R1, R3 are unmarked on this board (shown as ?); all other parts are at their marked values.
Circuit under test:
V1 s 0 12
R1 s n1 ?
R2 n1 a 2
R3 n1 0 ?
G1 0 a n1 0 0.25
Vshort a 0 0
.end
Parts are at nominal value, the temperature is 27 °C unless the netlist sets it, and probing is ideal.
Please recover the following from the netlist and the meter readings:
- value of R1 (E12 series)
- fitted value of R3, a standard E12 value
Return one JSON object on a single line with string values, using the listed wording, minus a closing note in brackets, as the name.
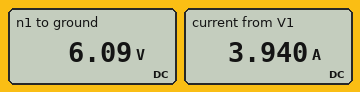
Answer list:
{"value of R1": "1.5 Ω", "fitted value of R3, a standard E12 value": "6.8 Ω"}
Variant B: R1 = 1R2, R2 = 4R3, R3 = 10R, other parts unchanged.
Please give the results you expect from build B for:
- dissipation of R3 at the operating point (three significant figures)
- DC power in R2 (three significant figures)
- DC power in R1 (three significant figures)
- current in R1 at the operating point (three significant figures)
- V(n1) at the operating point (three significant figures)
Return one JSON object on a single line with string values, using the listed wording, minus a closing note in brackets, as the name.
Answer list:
{"dissipation of R3 at the operating point": "7.36 W", "DC power in R2": "17.1 W", "DC power in R1": "9.76 W", "current in R1 at the operating point": "2.85 A", "V(n1) at the operating point": "8.58 V"}
